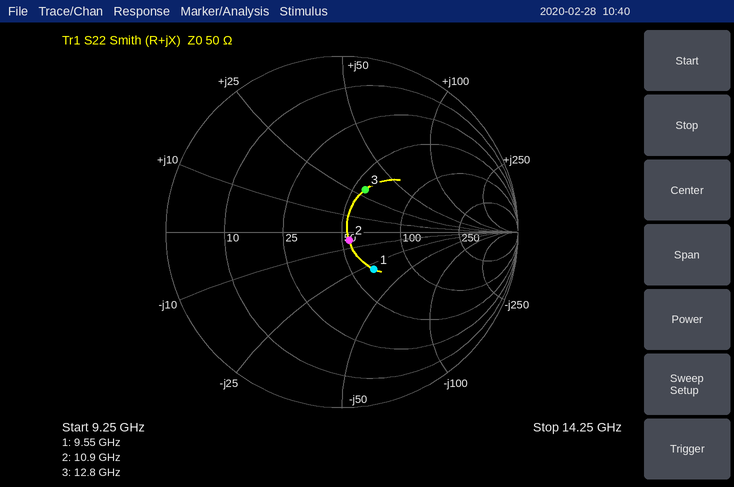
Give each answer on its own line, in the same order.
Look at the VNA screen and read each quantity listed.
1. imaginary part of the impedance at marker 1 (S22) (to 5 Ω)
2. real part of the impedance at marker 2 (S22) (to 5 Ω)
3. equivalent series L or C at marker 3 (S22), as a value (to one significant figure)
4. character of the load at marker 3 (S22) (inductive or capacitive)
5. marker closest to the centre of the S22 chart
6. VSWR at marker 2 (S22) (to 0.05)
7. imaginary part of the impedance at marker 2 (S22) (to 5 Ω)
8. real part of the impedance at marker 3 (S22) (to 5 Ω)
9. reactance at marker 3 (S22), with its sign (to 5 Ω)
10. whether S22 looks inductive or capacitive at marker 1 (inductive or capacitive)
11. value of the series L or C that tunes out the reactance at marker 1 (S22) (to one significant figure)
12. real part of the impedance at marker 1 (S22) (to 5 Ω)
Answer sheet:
-30 Ω
55 Ω
400 pH
inductive
marker 2
1.15
-5 Ω
55 Ω
+30 Ω
capacitive
500 pH
65 Ω
